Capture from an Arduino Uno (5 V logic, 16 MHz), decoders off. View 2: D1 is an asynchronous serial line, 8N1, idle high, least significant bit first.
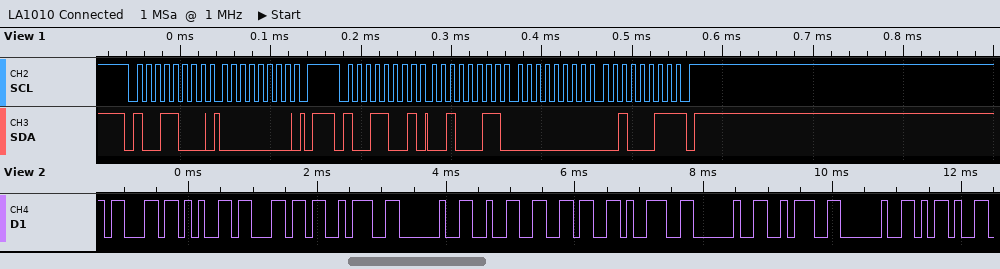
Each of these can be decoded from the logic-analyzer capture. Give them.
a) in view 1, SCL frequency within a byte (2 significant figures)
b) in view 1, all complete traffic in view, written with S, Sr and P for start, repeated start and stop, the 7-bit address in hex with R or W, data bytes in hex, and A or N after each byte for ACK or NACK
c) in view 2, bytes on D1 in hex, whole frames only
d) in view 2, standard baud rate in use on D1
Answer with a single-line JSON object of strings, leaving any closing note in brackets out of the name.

{"in view 1, SCL frequency within a byte": "100 kHz", "in view 1, all complete traffic in view, written with S, Sr and P for start, repeated start and stop, the 7-bit address in hex with R or W, data bytes in hex, and A or N after each byte for ACK or NACK": "S 4CW A 00 A P S 4CR A 23 A 00 A 23 N P", "in view 2, bytes on D1 in hex, whole frames only": "63 65 6C 3A 20 32 36 39 20 3A 20 2D", "in view 2, standard baud rate in use on D1": "9600 baud"}
